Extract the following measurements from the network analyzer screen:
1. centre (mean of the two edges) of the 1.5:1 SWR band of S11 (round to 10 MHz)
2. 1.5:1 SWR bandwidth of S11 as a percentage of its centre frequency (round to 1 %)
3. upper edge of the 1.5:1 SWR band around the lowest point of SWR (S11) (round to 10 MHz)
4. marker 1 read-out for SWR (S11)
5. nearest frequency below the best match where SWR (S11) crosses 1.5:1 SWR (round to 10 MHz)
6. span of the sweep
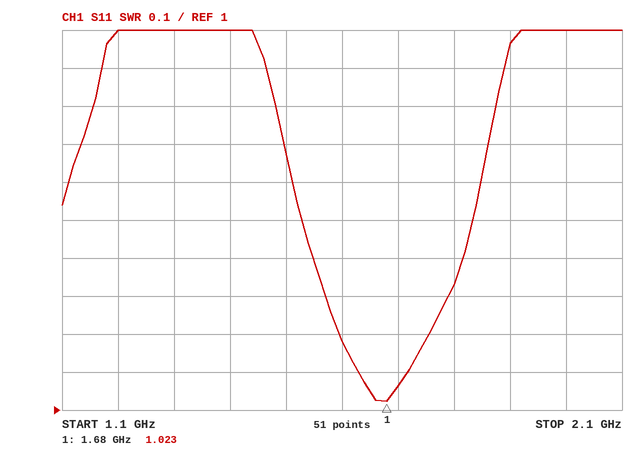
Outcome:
1.68 GHz
18 %
1.83 GHz
1.023
1.53 GHz
1 GHz
